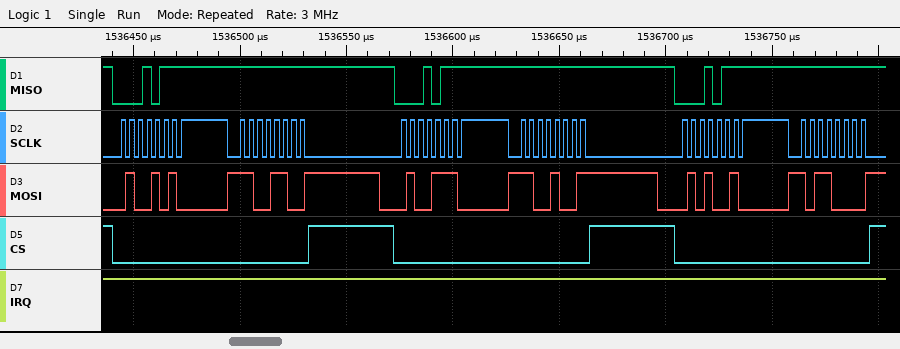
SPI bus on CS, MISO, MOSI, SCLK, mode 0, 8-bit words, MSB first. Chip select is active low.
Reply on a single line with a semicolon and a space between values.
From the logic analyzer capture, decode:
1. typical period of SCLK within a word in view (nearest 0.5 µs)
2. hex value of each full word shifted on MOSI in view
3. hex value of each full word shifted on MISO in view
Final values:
4 µs; 4A, CC, 4E, C9, 52, B0; 17, FF, 17, FF, 17, FF
